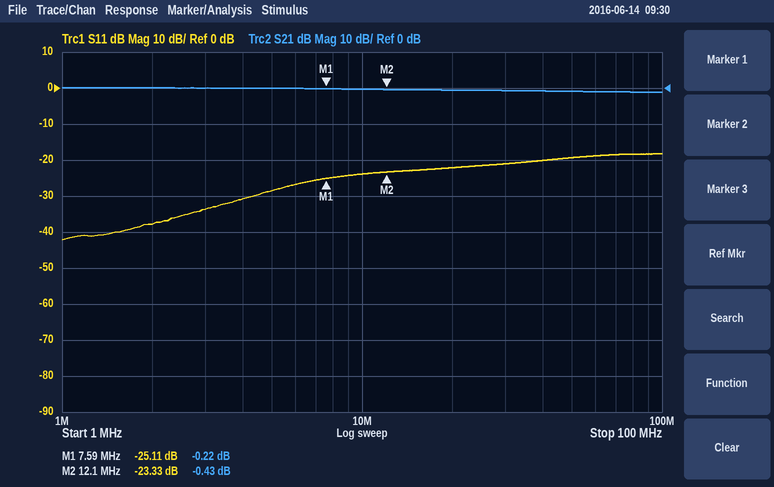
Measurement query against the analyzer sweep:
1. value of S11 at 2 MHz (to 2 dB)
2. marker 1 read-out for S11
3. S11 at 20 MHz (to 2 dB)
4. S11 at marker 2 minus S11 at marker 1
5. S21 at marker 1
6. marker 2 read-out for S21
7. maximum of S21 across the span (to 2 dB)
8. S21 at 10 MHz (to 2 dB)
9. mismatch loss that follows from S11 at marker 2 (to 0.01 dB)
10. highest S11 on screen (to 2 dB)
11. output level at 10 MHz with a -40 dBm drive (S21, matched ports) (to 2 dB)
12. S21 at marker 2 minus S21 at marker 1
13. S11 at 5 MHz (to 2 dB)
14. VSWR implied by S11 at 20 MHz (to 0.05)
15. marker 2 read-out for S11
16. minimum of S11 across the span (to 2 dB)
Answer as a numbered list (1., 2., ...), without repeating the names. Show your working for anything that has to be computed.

1. -38 dB
2. -25.11 dB
3. -22 dB
4. -23.33 − (-25.11) = 1.78 dB
5. -0.22 dB
6. -0.43 dB
7. 0 dB
8. 0 dB
9. −10 log10(1 − 10^(-23.33/10)) ≈ 0.02 dB
10. -18 dB
11. -40 dBm + (0 dB) = -40 dBm
12. -0.43 − (-0.22) = -0.21 dB
13. -28 dB
14. |Γ| = 10^(-22/20) = 0.0794; VSWR = (1 + 0.0794)/(1 − 0.0794) ≈ 1.17, so 1.15 to the nearest 0.05
15. -23.33 dB
16. -42 dB
